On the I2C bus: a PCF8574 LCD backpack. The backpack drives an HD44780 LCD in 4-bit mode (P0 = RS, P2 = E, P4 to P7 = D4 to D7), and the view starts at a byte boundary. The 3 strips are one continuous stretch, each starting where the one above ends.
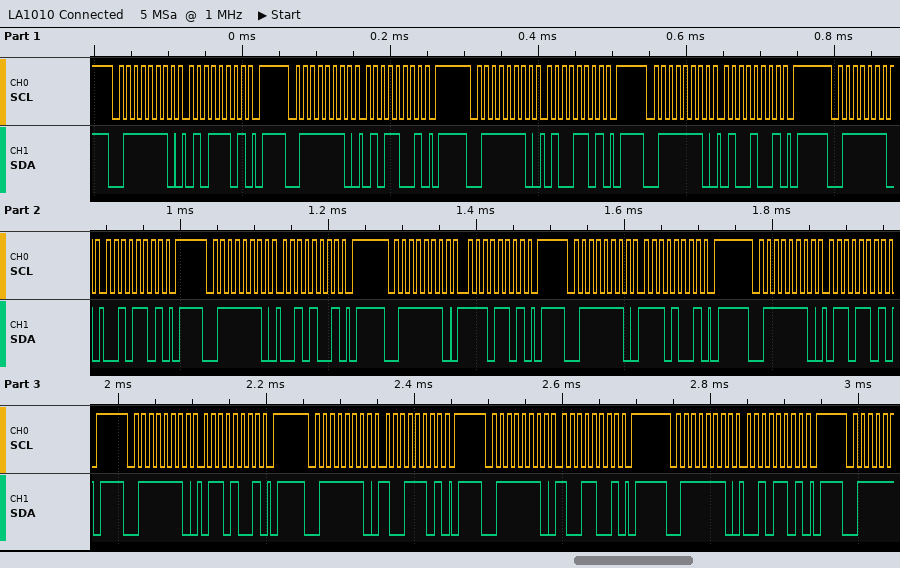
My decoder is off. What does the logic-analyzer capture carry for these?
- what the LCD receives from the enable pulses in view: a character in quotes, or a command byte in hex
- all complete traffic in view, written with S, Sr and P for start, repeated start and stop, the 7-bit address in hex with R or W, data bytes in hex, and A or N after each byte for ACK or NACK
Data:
'T' '.' 'i'
S 3FW A 5D A P S 3FW A 59 A P S 3FW A 4D A P S 3FW A 49 A P S 3FW A 2D A P S 3FW A 29 A P S 3FW A ED A P S 3FW A E9 A P S 3FW A 6D A P S 3FW A 69 A P S 3FW A 9D A P S 3FW A 99 A P S 3FW A 2D A P
